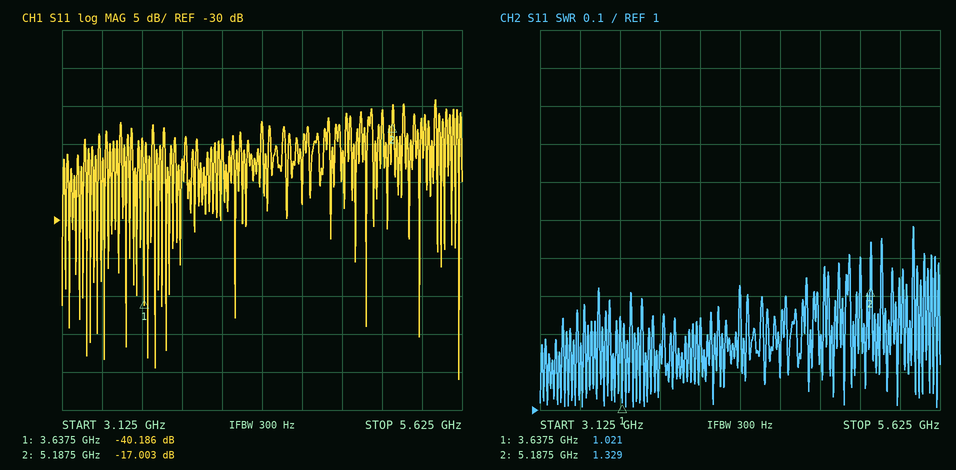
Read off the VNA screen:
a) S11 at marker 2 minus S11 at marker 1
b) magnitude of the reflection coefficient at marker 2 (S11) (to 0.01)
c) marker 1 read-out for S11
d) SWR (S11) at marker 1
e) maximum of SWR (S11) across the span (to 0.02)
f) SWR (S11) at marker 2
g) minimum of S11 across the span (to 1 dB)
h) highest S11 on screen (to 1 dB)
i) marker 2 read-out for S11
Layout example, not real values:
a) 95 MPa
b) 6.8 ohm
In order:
a) 23.183 dB
b) 0.14
c) -40.186 dB
d) 1.021
e) 1.48
f) 1.329
g) -51 dB
h) -14 dB
i) -17.003 dB
